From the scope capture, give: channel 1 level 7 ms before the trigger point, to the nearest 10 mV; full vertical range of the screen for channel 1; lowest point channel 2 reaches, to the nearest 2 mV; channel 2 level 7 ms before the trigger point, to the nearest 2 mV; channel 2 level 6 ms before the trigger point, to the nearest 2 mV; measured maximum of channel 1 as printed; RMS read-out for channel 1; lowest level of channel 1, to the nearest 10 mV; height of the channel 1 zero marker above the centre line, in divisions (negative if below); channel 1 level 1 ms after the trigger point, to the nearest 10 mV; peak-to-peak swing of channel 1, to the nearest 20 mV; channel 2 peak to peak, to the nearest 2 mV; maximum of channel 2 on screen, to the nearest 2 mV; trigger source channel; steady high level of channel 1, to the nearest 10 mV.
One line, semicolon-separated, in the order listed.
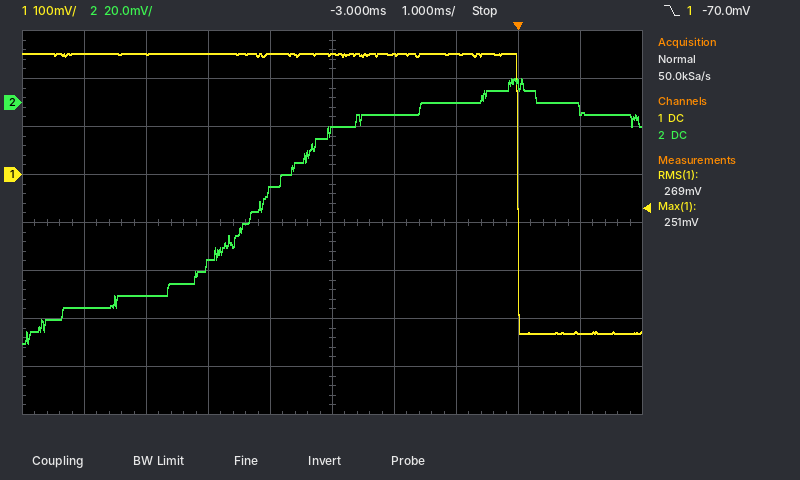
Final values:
250 mV; 800 mV; -100 mV; -86 mV; -80 mV; 251 mV; 269 mV; -330 mV; +1.0 div; -330 mV; 580 mV; 110 mV; 10 mV; channel 1; 250 mV
